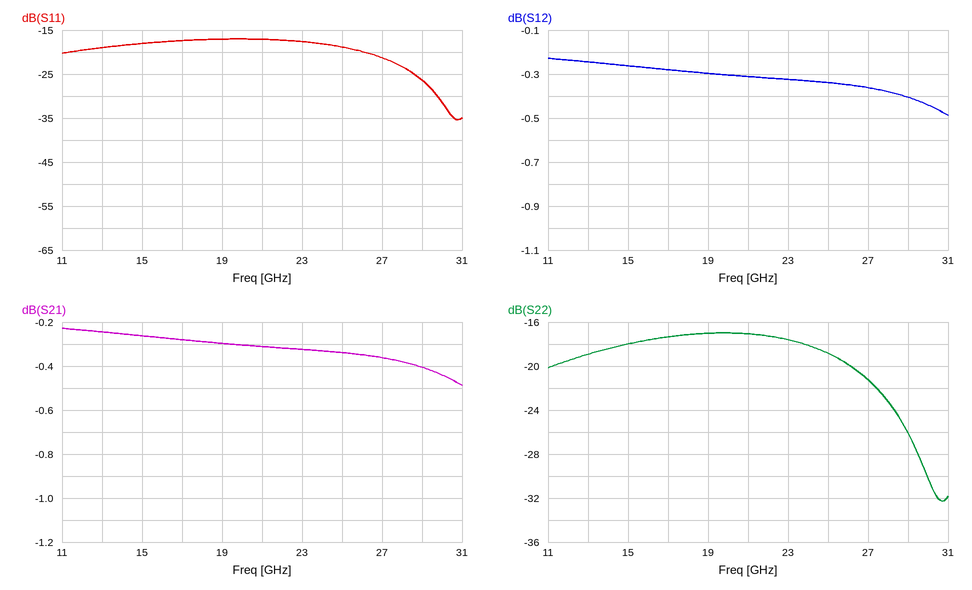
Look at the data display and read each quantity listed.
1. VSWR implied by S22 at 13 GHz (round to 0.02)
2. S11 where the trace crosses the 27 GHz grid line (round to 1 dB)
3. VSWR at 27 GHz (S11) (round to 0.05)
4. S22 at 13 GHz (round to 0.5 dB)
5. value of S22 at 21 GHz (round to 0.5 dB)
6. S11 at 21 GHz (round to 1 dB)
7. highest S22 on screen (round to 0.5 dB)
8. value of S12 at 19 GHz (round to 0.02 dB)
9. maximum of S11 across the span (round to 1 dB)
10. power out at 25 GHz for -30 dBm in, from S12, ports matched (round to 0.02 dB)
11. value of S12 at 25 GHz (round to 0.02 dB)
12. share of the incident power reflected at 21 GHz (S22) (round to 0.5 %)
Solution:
1.26
-21 dB
1.20
-19.0 dB
-17.0 dB
-17 dB
-17.0 dB
-0.30 dB
-17 dB
-30.34 dBm
-0.34 dB
2.0 %
